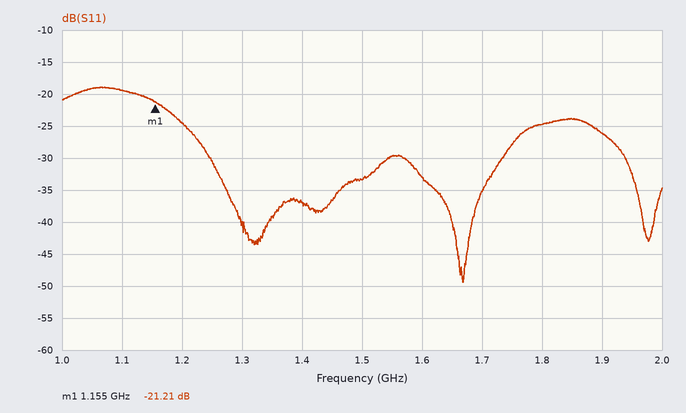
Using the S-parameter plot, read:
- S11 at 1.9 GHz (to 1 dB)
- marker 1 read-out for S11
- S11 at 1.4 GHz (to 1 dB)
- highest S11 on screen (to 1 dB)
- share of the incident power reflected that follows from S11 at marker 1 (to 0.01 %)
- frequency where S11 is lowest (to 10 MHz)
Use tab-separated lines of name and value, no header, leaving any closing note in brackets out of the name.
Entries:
S11 at 1.9 GHz	-26 dB
marker 1 read-out for S11	-21.21 dB
S11 at 1.4 GHz	-37 dB
highest S11 on screen	-19 dB
share of the incident power reflected that follows from S11 at marker 1	0.76 %
frequency where S11 is lowest	1.67 GHz
